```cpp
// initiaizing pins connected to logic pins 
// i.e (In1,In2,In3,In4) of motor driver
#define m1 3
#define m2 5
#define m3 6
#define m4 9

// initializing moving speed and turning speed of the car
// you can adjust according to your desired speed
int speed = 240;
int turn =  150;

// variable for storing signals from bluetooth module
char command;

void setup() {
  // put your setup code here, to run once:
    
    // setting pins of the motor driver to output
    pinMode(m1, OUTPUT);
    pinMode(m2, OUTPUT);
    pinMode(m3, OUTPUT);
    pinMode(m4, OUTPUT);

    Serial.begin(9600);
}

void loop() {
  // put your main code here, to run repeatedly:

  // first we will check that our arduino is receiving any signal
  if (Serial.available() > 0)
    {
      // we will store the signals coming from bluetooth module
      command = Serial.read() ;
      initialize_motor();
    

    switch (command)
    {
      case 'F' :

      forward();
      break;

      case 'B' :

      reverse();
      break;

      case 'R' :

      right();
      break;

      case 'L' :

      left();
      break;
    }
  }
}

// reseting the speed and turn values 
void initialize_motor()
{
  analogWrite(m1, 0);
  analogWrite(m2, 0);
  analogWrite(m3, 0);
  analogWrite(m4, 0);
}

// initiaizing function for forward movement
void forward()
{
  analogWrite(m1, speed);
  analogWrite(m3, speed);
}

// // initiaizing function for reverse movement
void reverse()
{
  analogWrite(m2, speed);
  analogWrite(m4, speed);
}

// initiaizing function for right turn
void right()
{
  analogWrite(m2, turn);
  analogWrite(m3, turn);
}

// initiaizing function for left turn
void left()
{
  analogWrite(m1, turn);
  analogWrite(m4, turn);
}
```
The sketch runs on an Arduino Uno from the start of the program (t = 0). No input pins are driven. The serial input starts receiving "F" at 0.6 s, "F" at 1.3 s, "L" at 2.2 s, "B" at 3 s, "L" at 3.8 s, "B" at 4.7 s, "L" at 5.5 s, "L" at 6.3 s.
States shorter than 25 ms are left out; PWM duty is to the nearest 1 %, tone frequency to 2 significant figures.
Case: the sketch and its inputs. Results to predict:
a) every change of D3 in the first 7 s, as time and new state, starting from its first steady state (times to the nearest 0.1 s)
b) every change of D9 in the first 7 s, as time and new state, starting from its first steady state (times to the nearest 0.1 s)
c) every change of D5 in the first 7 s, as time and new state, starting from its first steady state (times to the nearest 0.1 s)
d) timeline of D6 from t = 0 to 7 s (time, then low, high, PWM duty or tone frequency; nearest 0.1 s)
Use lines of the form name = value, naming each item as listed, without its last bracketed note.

every change of D3 in the first 7 s, as time and new state, starting from its first steady state = 0 s low; 0.6 s PWM 94 %; 2.2 s PWM 59 %; 3 s low; 3.8 s PWM 59 %; 4.7 s low; 5.5 s PWM 59 %
every change of D9 in the first 7 s, as time and new state, starting from its first steady state = 0 s low; 2.2 s PWM 59 %; 3 s PWM 94 %; 3.8 s PWM 59 %; 4.7 s PWM 94 %; 5.5 s PWM 59 %
every change of D5 in the first 7 s, as time and new state, starting from its first steady state = 0 s low; 3 s PWM 94 %; 3.8 s low; 4.7 s PWM 94 %; 5.5 s low
timeline of D6 from t = 0 to 7 s = 0 s low; 0.6 s PWM 94 %; 2.2 s low
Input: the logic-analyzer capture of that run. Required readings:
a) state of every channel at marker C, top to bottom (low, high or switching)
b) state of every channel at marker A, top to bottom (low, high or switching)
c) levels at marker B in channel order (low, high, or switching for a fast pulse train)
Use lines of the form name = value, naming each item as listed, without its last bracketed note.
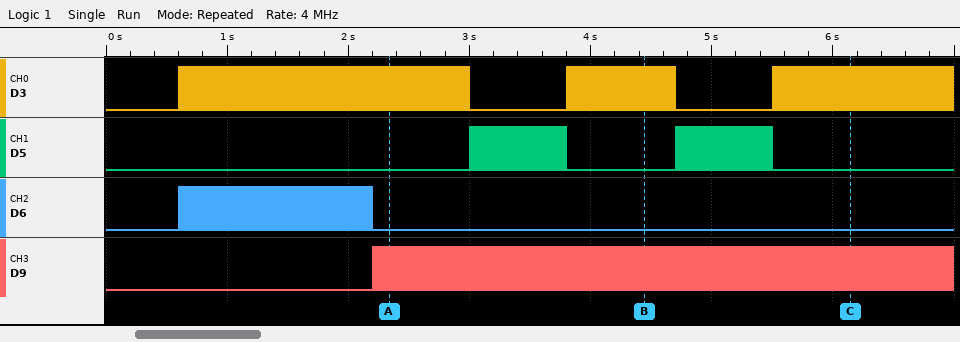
state of every channel at marker C, top to bottom = D3 switching, D5 low, D6 low, D9 switching
state of every channel at marker A, top to bottom = D3 switching, D5 low, D6 low, D9 switching
levels at marker B in channel order = D3 switching, D5 low, D6 low, D9 switching
